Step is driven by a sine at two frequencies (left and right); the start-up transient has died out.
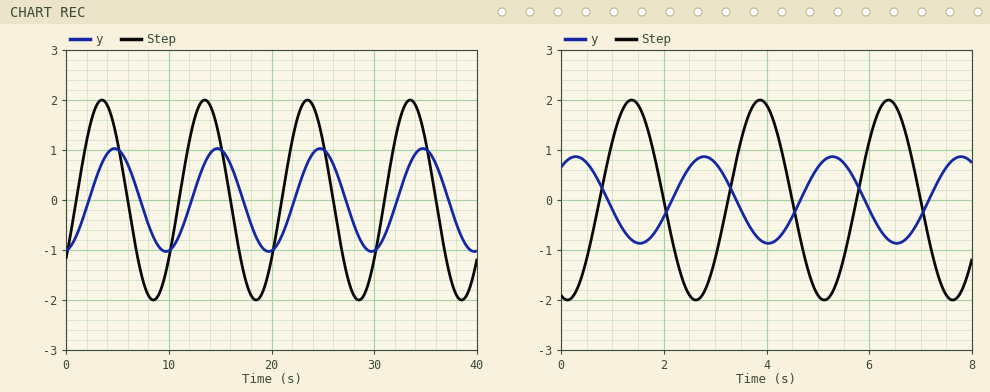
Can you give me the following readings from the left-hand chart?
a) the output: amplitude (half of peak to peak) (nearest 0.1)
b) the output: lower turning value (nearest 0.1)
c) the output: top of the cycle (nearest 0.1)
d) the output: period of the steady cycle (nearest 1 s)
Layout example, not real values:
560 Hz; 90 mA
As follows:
1.0; -1.0; 1.0; 10 s
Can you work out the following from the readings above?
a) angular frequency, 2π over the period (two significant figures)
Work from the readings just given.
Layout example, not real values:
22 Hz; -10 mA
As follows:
0.63 rad/s
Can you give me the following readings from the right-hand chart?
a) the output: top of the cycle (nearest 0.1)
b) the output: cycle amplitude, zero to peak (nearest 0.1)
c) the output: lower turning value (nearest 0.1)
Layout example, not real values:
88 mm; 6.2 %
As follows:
0.9; 0.9; -0.9
